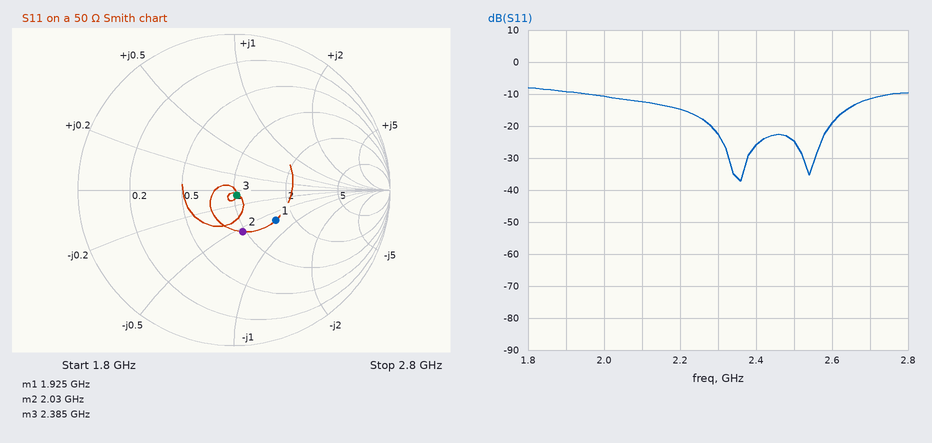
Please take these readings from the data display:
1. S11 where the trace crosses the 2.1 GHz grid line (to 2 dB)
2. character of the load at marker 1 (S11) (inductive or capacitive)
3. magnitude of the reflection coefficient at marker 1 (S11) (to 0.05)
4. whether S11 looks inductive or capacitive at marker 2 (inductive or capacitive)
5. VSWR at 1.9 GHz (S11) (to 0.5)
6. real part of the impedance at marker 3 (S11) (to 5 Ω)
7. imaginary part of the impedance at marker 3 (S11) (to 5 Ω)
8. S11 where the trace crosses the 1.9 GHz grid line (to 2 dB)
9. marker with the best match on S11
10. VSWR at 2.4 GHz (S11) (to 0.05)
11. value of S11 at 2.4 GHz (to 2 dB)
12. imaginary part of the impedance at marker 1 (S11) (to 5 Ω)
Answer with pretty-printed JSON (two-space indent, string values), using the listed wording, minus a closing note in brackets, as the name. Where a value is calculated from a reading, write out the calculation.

{
  "S11 where the trace crosses the 2.1 GHz grid line": "-12 dB",
  "character of the load at marker 1 (S11)": "capacitive",
  "magnitude of the reflection coefficient at marker 1 (S11)": "0.35",
  "whether S11 looks inductive or capacitive at marker 2": "capacitive",
  "VSWR at 1.9 GHz (S11)": "|Γ| = 10^(-10/20) = 0.3162; VSWR = (1 + 0.3162)/(1 − 0.3162) ≈ 1.92, so 2.0 to the nearest 0.5",
  "real part of the impedance at marker 3 (S11)": "50 Ω",
  "imaginary part of the impedance at marker 3 (S11)": "-5 Ω",
  "S11 where the trace crosses the 1.9 GHz grid line": "-10 dB",
  "marker with the best match on S11": "marker 3",
  "VSWR at 2.4 GHz (S11)": "|Γ| = 10^(-26/20) = 0.0501; VSWR = (1 + 0.0501)/(1 − 0.0501) ≈ 1.11, so 1.10 to the nearest 0.05",
  "value of S11 at 2.4 GHz": "-26 dB",
  "imaginary part of the impedance at marker 1 (S11)": "-35 Ω"
}
